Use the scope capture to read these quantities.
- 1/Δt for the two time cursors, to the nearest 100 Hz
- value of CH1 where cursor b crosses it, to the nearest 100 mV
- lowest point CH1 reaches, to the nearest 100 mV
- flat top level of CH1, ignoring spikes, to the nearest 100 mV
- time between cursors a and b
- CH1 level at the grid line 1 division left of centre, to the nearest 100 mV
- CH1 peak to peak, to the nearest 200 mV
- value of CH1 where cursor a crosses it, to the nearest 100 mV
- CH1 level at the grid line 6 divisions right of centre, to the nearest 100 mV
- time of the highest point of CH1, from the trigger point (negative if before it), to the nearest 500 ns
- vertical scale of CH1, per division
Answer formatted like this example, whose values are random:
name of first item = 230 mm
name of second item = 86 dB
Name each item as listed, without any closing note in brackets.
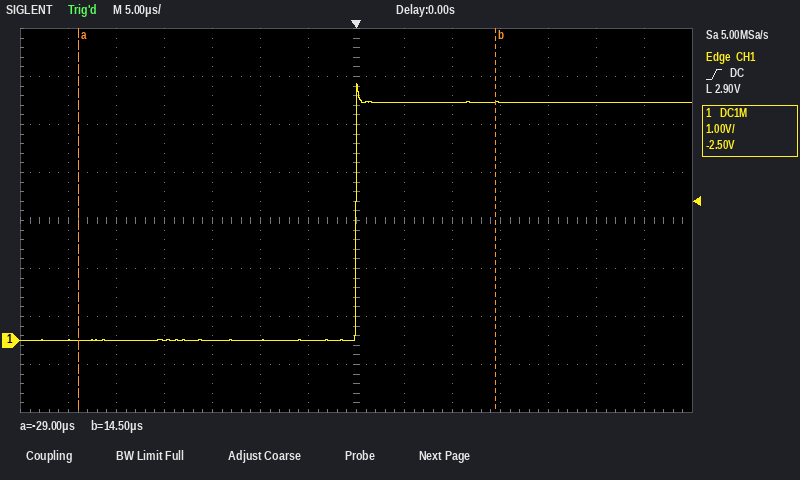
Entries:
1/Δt for the two time cursors, to the nearest 100 Hz = 23.0 kHz
value of CH1 where cursor b crosses it, to the nearest 100 mV = 5.0 V
lowest point CH1 reaches, to the nearest 100 mV = 0.0 V
flat top level of CH1, ignoring spikes, to the nearest 100 mV = 5.0 V
time between cursors a and b = 43.5 µs
CH1 level at the grid line 1 division left of centre, to the nearest 100 mV = 0.0 V
CH1 peak to peak, to the nearest 200 mV = 5.4 V
value of CH1 where cursor a crosses it, to the nearest 100 mV = 0.0 V
CH1 level at the grid line 6 divisions right of centre, to the nearest 100 mV = 5.0 V
time of the highest point of CH1, from the trigger point (negative if before it), to the nearest 500 ns = 0.0 µs
vertical scale of CH1, per division = 1 V
